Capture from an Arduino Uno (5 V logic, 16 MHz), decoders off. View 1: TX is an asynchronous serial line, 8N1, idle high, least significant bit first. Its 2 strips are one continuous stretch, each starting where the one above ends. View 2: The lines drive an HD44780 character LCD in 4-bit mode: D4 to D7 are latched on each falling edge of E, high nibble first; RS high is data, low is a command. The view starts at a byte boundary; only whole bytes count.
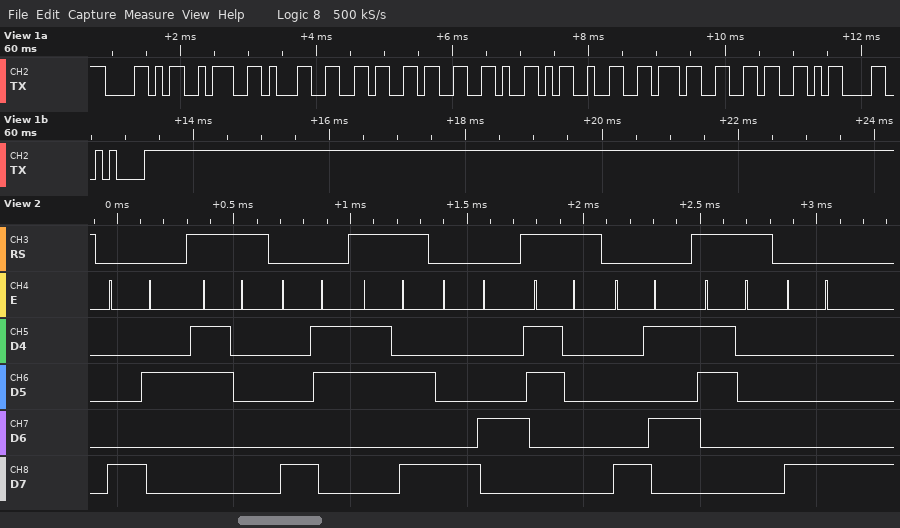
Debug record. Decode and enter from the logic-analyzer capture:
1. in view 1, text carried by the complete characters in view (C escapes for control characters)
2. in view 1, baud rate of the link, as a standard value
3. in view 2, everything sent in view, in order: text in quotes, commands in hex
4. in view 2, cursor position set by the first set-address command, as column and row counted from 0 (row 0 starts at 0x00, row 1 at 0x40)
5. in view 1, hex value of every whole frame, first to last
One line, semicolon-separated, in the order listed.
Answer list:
"X:163Y276\r\n"; 9600 baud; 0x82 "0" 0x83 ":" 0x84 "0" 0x85 "0" 0x88; column 2, row 0; 0x58 0x3A 0x31 0x36 0x33 0x59 0x32 0x37 0x36 0x0D 0x0A
